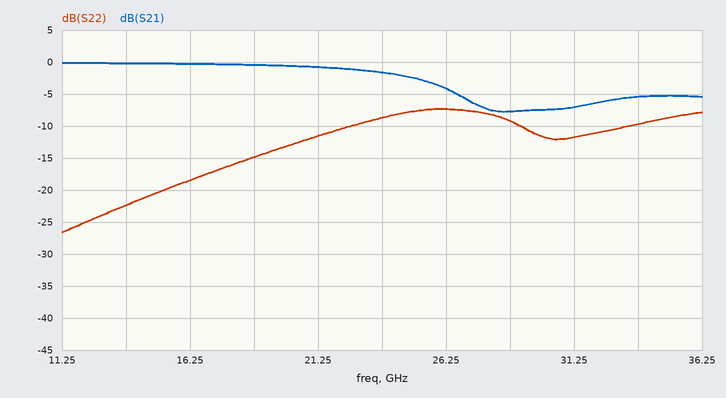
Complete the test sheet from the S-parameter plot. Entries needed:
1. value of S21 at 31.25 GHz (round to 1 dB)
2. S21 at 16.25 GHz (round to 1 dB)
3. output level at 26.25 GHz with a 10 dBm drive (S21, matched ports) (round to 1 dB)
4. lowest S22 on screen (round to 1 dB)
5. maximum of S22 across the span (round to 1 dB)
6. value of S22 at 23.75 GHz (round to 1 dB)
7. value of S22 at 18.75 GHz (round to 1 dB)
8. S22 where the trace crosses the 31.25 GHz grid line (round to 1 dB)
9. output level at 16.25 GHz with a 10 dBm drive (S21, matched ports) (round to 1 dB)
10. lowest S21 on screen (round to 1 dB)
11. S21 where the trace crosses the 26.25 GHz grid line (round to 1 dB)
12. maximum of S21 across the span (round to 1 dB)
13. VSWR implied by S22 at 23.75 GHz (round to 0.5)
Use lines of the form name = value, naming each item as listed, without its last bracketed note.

value of S21 at 31.25 GHz = -7 dB
S21 at 16.25 GHz = 0 dB
output level at 26.25 GHz with a 10 dBm drive (S21, matched ports) = 6 dBm
lowest S22 on screen = -27 dB
maximum of S22 across the span = -7 dB
value of S22 at 23.75 GHz = -9 dB
value of S22 at 18.75 GHz = -15 dB
S22 where the trace crosses the 31.25 GHz grid line = -12 dB
output level at 16.25 GHz with a 10 dBm drive (S21, matched ports) = 10 dBm
lowest S21 on screen = -8 dB
S21 where the trace crosses the 26.25 GHz grid line = -4 dB
maximum of S21 across the span = 0 dB
VSWR implied by S22 at 23.75 GHz = 2.0
